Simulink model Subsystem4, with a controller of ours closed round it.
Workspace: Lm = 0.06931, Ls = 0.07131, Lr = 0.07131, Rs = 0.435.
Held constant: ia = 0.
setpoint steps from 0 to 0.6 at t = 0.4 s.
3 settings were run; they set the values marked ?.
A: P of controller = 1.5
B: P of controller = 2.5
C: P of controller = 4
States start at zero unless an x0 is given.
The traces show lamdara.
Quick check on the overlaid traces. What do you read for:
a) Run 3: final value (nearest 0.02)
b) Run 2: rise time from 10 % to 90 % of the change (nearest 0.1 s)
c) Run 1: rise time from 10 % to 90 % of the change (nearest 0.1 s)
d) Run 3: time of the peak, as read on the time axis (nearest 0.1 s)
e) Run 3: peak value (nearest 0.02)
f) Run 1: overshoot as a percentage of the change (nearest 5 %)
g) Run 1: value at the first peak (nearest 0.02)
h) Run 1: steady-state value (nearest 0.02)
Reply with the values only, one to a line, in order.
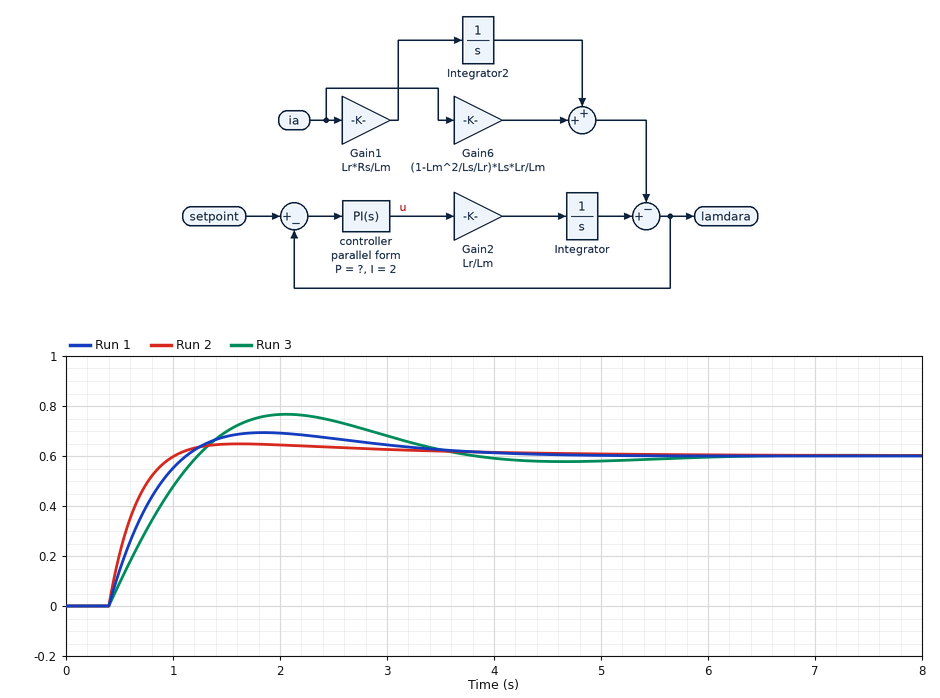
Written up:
0.60
0.4 s
0.5 s
2.1 s
0.76
15 %
0.70
0.60
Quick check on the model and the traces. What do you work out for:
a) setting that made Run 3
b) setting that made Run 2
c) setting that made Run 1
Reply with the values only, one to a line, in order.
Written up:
A
C
B
